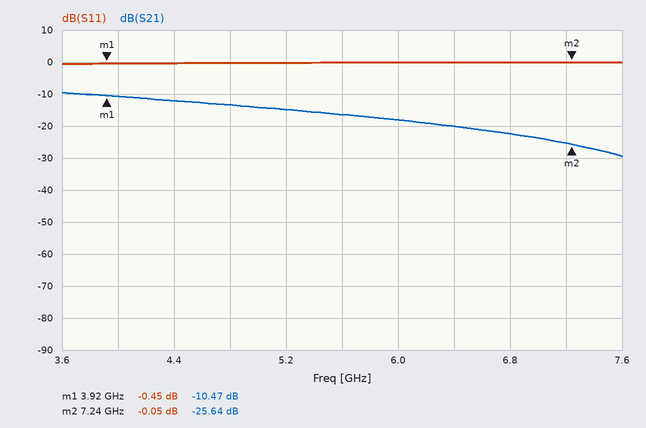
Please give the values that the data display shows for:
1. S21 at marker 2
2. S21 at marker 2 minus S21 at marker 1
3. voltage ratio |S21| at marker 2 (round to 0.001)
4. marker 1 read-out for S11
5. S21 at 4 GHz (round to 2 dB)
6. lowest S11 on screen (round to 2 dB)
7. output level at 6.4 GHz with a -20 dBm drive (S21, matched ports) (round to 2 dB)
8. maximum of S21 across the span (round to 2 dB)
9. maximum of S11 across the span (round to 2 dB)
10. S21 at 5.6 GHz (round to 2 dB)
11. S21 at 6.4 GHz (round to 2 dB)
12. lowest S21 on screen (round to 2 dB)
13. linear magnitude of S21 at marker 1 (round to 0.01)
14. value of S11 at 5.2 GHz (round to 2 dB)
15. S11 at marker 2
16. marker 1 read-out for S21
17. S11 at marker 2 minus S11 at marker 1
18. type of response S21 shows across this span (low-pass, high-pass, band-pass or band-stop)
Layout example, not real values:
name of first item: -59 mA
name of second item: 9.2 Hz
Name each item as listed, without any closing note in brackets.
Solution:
S21 at marker 2: -25.64 dB
S21 at marker 2 minus S21 at marker 1: -15.17 dB
voltage ratio |S21| at marker 2: 0.052
marker 1 read-out for S11: -0.45 dB
S21 at 4 GHz: -10 dB
lowest S11 on screen: 0 dB
output level at 6.4 GHz with a -20 dBm drive (S21, matched ports): -40 dBm
maximum of S21 across the span: -10 dB
maximum of S11 across the span: 0 dB
S21 at 5.6 GHz: -16 dB
S21 at 6.4 GHz: -20 dB
lowest S21 on screen: -30 dB
linear magnitude of S21 at marker 1: 0.30
value of S11 at 5.2 GHz: 0 dB
S11 at marker 2: -0.05 dB
marker 1 read-out for S21: -10.47 dB
S11 at marker 2 minus S11 at marker 1: 0.40 dB
type of response S21 shows across this span: low-pass
